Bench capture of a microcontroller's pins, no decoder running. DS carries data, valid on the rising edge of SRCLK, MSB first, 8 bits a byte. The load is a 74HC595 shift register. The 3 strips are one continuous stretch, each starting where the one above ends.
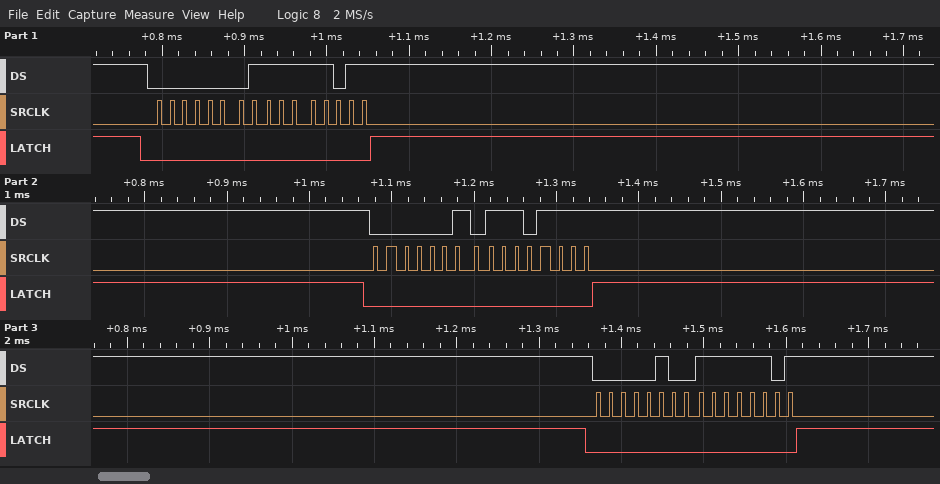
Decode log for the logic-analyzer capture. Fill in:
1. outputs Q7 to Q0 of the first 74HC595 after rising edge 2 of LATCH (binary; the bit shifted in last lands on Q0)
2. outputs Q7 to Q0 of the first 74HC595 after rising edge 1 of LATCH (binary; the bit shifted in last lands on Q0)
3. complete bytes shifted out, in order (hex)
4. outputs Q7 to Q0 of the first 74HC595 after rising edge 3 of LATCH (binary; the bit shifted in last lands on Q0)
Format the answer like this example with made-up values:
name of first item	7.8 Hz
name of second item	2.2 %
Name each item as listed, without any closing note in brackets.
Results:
outputs Q7 to Q0 of the first 74HC595 after rising edge 2 of LATCH	11101111
outputs Q7 to Q0 of the first 74HC595 after rising edge 1 of LATCH	11111011
complete bytes shifted out, in order	01 FB 02 EF 04 FD
outputs Q7 to Q0 of the first 74HC595 after rising edge 3 of LATCH	11111101
